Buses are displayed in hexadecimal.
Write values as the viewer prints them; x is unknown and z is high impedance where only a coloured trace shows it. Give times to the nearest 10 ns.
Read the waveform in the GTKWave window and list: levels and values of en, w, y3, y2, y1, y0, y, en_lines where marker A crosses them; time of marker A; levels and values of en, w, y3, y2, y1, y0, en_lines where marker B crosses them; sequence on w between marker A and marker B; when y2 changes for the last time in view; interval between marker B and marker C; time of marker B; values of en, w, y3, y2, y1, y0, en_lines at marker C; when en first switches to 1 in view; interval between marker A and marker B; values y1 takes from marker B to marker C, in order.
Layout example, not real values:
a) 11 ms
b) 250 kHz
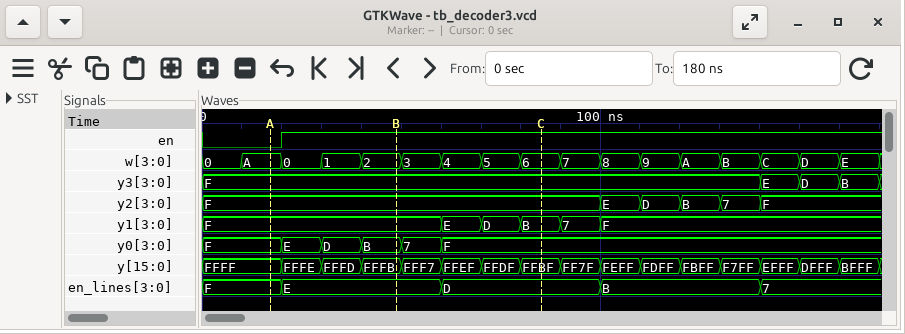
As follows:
a) en=0, w=A, y3=F, y2=F, y1=F, y0=F, y=FFFF, en_lines=F
b) 20 ns
c) en=1, w=2, y3=F, y2=F, y1=F, y0=B, en_lines=E
d) A, 0, 1, 2
e) 140 ns
f) 40 ns
g) 50 ns
h) en=1, w=6, y3=F, y2=F, y1=B, y0=F, en_lines=D
i) 20 ns
j) 30 ns
k) F, E, D, B
